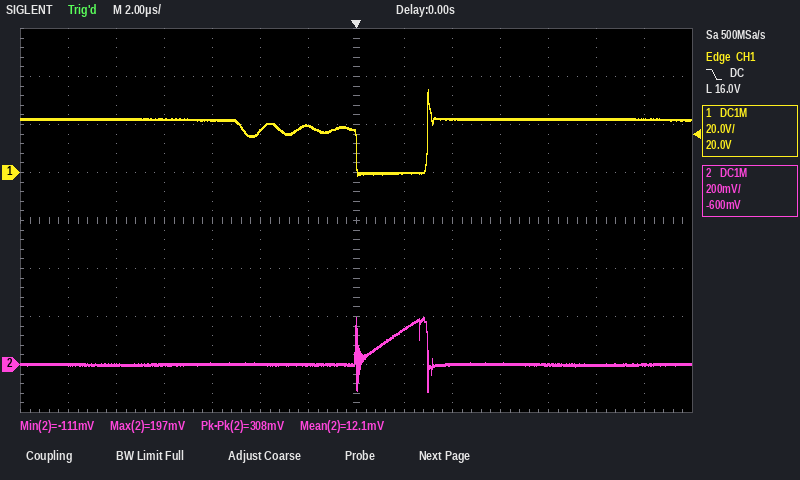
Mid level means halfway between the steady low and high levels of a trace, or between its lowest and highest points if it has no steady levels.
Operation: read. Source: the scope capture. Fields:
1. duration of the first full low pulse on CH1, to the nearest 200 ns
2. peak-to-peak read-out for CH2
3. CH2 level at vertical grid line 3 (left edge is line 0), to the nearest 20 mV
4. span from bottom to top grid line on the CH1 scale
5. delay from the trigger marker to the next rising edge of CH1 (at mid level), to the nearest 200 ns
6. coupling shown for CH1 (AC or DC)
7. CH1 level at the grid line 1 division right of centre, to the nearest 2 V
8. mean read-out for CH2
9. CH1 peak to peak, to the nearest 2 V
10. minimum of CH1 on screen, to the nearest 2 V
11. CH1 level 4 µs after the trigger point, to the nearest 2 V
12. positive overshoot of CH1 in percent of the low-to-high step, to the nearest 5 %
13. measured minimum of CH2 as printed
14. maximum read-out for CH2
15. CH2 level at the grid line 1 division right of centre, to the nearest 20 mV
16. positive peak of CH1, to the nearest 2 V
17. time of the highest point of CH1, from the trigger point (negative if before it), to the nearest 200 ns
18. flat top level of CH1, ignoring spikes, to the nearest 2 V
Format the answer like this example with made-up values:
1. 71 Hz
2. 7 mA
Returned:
1. 3.0 µs
2. 308 mV
3. 0 mV
4. 160 V
5. 3.0 µs
6. DC
7. 0 V
8. 12.1 mV
9. 36 V
10. -2 V
11. 22 V
12. 55 %
13. -111 mV
14. 197 mV
15. 140 mV
16. 34 V
17. +3.0 µs
18. 22 V
